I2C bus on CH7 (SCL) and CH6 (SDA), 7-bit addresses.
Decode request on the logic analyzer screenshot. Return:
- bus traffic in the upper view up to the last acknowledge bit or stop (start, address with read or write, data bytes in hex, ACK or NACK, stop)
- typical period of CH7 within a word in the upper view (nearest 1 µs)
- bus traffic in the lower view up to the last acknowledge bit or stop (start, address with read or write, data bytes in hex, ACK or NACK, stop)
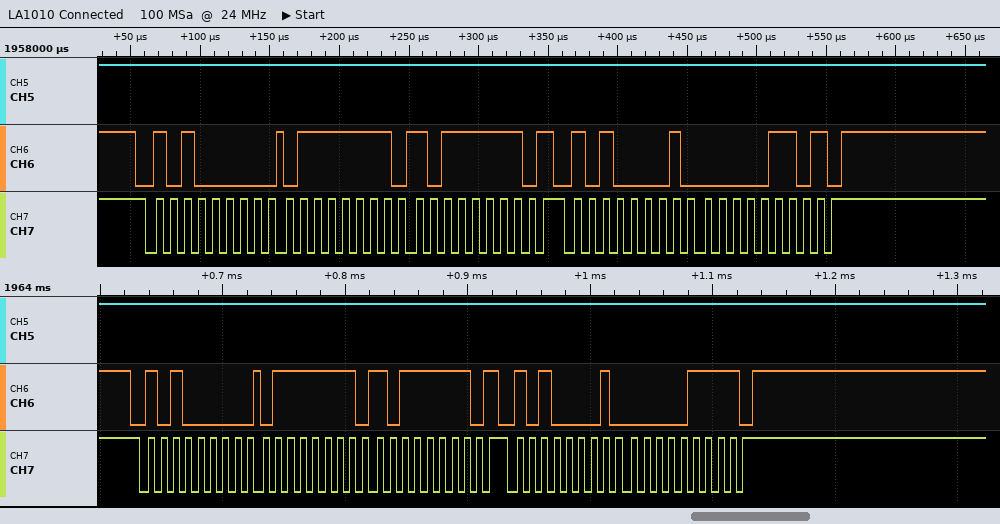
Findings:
start, address 50 write ACK, 7F ACK, BF ACK, repeated start, address 50 read ACK, 06 NACK, stop
10 µs
start, address 50 write ACK, 7F ACK, BF ACK, repeated start, address 50 read ACK, 07 NACK, stop
